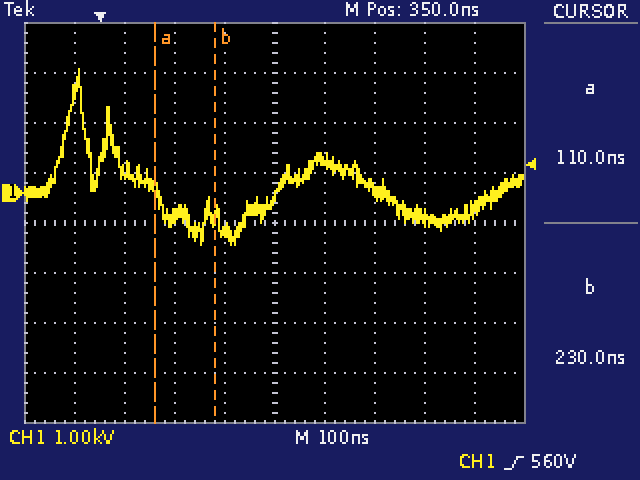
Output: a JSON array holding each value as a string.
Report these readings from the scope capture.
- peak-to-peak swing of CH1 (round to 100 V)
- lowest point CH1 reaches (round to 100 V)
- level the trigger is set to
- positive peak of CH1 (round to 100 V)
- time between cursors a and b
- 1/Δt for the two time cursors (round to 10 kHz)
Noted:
["3.5 kV", "-1.0 kV", "560 V", "2.5 kV", "120 ns", "8.33 MHz"]
